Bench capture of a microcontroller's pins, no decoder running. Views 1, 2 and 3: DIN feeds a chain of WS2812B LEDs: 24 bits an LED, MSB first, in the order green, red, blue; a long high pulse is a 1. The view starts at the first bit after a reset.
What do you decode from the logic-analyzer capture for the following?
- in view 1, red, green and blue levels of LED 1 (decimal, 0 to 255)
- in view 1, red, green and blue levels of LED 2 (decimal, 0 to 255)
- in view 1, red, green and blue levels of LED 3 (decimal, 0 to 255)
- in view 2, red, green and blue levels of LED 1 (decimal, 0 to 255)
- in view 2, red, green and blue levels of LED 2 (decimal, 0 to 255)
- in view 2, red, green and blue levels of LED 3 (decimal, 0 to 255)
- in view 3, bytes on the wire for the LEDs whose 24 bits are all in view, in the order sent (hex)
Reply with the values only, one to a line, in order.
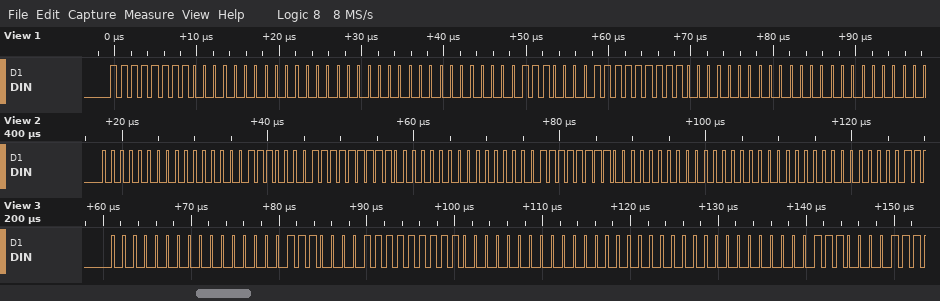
0, 255, 0
0, 0, 225
0, 255, 0
0, 0, 225
0, 255, 0
0, 255, 0
00 00 E1 FF 00 00 00 00 E1
